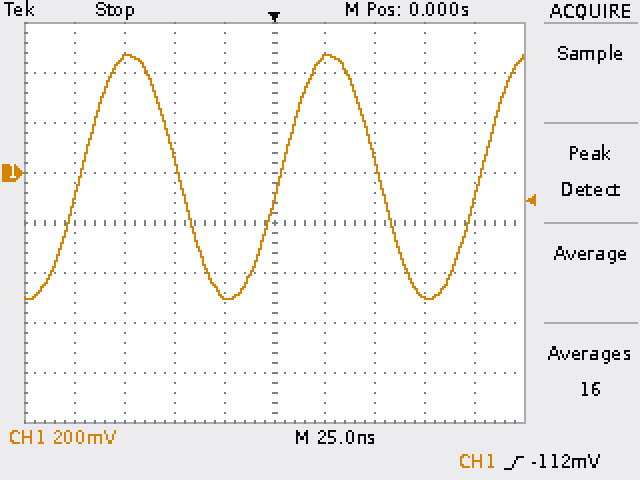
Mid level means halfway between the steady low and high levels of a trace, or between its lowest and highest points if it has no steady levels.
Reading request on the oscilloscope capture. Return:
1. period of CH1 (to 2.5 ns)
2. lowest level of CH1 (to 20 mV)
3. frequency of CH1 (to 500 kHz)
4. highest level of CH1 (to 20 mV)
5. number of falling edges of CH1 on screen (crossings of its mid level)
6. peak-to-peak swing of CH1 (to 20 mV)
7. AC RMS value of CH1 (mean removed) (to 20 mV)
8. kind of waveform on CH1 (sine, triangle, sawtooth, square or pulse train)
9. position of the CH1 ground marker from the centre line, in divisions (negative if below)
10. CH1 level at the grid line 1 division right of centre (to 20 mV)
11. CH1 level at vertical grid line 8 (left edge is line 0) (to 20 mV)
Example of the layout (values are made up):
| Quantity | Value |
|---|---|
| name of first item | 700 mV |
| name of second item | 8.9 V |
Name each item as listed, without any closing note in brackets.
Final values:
| Quantity | Value |
|---|---|
| period of CH1 | 100.0 ns |
| lowest level of CH1 | -500 mV |
| frequency of CH1 | 10.0 MHz |
| highest level of CH1 | 480 mV |
| number of falling edges of CH1 on screen | 2 |
| peak-to-peak swing of CH1 | 980 mV |
| AC RMS value of CH1 (mean removed) | 340 mV |
| kind of waveform on CH1 | sine |
| position of the CH1 ground marker from the centre line, in divisions | +1.0 div |
| CH1 level at the grid line 1 division right of centre | 460 mV |
| CH1 level at vertical grid line 8 (left edge is line 0) | -500 mV |
